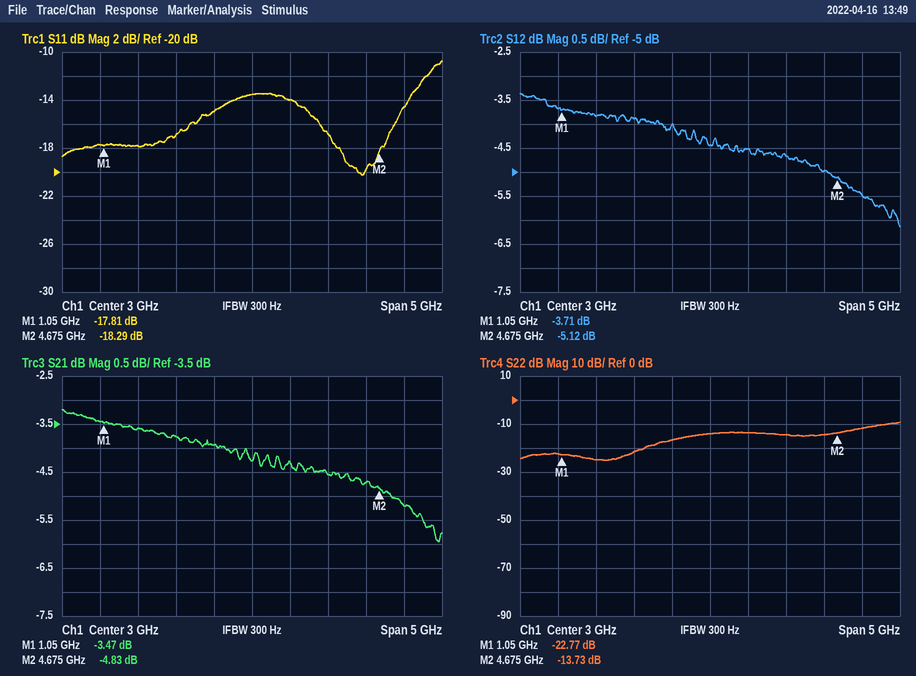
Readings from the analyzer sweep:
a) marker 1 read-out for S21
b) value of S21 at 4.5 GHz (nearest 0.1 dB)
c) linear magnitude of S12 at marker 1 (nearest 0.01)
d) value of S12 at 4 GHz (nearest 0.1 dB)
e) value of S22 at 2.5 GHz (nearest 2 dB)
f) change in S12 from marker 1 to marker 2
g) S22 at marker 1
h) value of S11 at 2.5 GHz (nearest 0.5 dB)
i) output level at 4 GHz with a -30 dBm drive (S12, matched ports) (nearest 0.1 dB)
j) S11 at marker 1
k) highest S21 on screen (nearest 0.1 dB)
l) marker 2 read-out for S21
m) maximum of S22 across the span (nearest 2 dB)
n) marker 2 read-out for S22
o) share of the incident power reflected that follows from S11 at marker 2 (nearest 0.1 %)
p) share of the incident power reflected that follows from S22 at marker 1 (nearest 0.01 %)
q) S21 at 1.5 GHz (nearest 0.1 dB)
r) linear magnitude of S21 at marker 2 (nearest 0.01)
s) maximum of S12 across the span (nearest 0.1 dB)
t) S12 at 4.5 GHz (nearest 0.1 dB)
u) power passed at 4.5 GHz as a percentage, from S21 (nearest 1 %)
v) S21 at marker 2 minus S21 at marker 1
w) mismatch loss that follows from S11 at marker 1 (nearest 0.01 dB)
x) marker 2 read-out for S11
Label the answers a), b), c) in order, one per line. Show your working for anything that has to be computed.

a) -3.47 dB
b) -4.7 dB
c) 10^(-3.71/20) ≈ 0.65
d) -4.7 dB
e) -16 dB
f) -5.12 − (-3.71) = -1.41 dB
g) -22.77 dB
h) -15.0 dB
i) -30 dBm + (-4.7 dB) = -34.7 dBm
j) -17.81 dB
k) -3.2 dB
l) -4.83 dB
m) -10 dB
n) -13.73 dB
o) 10^(-18.29/10) ≈ 1.5 %
p) 10^(-22.77/10) ≈ 0.53 %
q) -3.6 dB
r) 10^(-4.83/20) ≈ 0.57
s) -3.4 dB
t) -5.0 dB
u) 10^(-4.7/10) ≈ 34 %
v) -4.83 − (-3.47) = -1.36 dB
w) −10 log10(1 − 10^(-17.81/10)) ≈ 0.07 dB
x) -18.29 dB
